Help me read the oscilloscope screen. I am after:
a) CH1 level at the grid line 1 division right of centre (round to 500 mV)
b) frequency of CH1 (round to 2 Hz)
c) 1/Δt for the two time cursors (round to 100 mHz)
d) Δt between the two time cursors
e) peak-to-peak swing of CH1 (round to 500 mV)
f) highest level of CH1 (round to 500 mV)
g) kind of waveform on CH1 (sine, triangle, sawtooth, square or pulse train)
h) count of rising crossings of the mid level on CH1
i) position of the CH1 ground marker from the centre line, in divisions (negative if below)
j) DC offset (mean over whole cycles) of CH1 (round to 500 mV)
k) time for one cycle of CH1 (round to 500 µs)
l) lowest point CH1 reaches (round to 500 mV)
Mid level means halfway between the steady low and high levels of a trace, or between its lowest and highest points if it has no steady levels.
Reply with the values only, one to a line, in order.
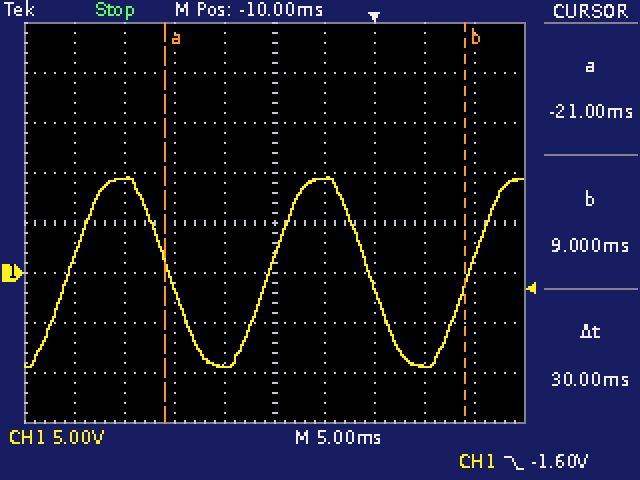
9.5 V
50 Hz
33.3 Hz
30 ms
19.0 V
9.5 V
sine
3
-1.0 div
0.0 V
20.0 ms
-9.5 V
